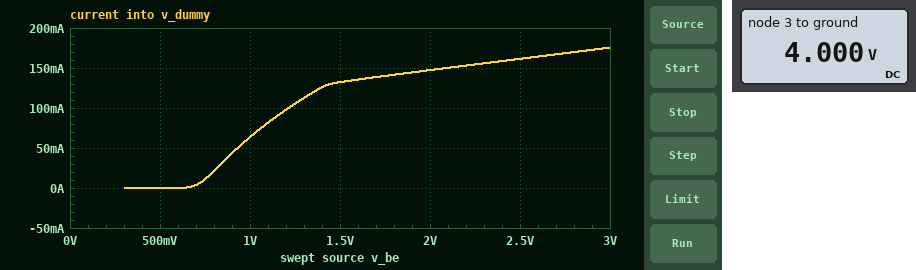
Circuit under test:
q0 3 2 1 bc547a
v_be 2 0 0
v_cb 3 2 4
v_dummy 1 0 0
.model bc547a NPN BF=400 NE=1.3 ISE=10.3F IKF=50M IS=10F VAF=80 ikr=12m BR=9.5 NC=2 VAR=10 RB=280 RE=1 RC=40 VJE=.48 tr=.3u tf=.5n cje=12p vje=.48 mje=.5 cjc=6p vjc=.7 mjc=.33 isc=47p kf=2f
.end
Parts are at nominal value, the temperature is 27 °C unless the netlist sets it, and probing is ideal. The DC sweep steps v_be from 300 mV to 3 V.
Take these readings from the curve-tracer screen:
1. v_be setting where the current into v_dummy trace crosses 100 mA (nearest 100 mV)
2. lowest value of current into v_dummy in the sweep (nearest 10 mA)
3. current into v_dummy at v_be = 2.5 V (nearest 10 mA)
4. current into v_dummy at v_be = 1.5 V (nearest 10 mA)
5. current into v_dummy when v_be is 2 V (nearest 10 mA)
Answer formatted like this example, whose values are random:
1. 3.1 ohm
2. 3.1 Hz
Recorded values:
1. 1.2 V
2. 0 A
3. 160 mA
4. 130 mA
5. 150 mA
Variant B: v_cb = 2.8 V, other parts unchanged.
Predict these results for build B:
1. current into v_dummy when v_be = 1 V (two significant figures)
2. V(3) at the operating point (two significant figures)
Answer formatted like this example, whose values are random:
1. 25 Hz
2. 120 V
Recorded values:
1. 63 mA
2. 2.8 V
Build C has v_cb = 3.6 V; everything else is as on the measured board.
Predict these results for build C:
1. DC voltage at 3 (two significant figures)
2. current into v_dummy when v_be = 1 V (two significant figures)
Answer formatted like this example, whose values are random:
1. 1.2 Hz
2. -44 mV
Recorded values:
1. 3.6 V
2. 63 mA
